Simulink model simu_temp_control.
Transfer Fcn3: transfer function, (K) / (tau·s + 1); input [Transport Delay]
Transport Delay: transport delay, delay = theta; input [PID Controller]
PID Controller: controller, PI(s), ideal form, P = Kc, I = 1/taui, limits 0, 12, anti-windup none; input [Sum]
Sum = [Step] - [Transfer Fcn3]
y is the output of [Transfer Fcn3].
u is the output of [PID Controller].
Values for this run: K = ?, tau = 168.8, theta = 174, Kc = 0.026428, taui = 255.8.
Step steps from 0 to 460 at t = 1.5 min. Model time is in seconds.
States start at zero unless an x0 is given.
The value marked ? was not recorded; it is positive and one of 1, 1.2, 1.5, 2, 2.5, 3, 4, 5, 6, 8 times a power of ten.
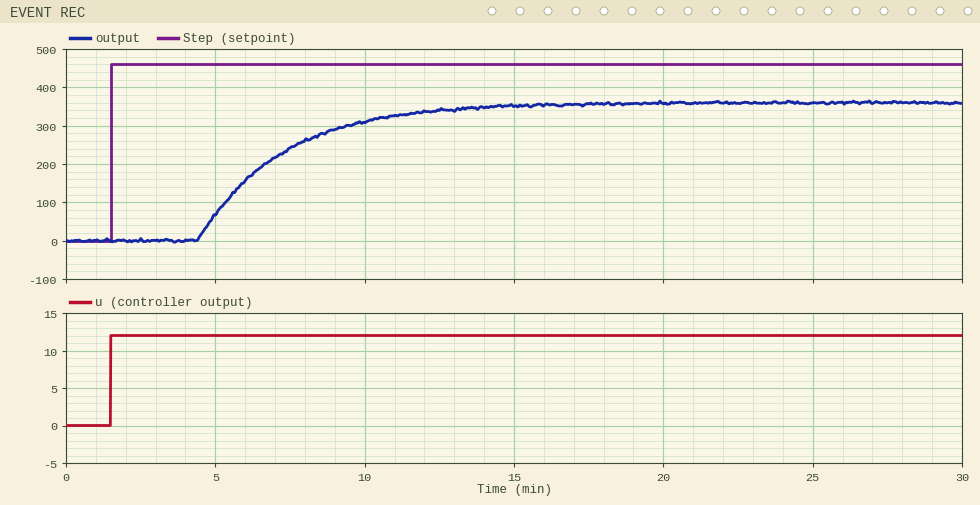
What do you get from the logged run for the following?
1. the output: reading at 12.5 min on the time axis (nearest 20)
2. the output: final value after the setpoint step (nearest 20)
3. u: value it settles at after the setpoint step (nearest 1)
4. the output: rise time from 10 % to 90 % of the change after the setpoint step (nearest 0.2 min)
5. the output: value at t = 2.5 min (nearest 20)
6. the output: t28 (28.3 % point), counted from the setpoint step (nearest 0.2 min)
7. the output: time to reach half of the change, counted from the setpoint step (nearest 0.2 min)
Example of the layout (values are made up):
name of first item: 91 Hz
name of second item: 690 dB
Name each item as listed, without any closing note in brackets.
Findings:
the output: reading at 12.5 min on the time axis: 340
the output: final value after the setpoint step: 360
u: value it settles at after the setpoint step: 12
the output: rise time from 10 % to 90 % of the change after the setpoint step: 6.2 min
the output: value at t = 2.5 min: 0
the output: t28 (28.3 % point), counted from the setpoint step: 3.8 min
the output: time to reach half of the change, counted from the setpoint step: 4.8 min
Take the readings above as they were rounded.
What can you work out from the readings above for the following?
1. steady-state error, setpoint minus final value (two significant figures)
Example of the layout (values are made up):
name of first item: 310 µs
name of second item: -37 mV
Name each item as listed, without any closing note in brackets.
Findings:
steady-state error, setpoint minus final value: 100
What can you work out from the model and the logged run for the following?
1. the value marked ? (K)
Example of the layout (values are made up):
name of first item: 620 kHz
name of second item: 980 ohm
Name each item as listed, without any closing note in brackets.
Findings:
the value marked ?: 30
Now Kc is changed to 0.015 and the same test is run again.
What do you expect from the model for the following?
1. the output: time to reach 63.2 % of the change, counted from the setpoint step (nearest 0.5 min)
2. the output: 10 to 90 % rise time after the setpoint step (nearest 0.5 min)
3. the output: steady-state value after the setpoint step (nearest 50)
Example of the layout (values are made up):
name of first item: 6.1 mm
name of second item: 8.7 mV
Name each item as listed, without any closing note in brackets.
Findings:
the output: time to reach 63.2 % of the change, counted from the setpoint step: 6.5 min
the output: 10 to 90 % rise time after the setpoint step: 7.0 min
the output: steady-state value after the setpoint step: 350
